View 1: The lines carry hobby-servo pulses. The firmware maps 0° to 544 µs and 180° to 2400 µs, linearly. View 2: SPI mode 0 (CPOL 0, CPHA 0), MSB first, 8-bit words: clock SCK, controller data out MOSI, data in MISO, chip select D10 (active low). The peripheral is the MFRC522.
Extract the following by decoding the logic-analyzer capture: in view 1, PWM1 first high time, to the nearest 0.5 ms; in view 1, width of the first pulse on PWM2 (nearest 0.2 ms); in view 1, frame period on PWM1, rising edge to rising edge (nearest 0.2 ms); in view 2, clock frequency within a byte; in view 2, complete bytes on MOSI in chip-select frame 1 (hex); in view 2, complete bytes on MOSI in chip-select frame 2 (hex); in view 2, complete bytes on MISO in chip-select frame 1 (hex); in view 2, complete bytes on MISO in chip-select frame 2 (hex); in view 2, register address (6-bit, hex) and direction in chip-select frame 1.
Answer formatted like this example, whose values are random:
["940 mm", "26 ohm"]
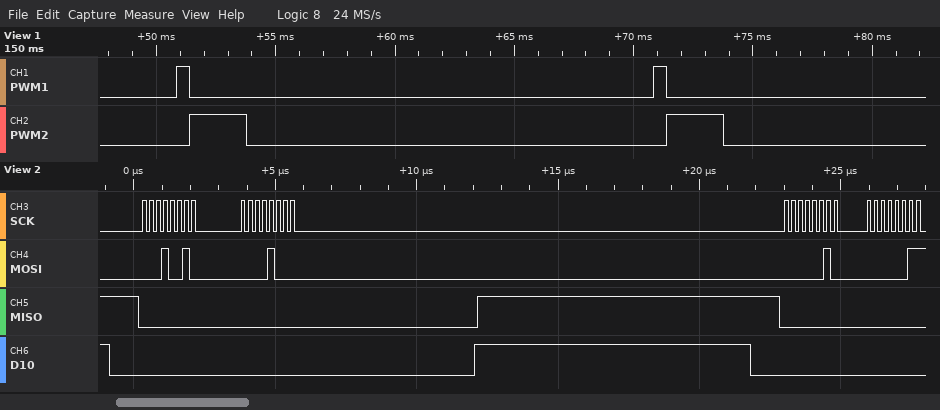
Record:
["0.5 ms", "2.4 ms", "20.0 ms", "4 MHz", "12 08", "02 03", "00 00", "00 00", "0x09 write"]
